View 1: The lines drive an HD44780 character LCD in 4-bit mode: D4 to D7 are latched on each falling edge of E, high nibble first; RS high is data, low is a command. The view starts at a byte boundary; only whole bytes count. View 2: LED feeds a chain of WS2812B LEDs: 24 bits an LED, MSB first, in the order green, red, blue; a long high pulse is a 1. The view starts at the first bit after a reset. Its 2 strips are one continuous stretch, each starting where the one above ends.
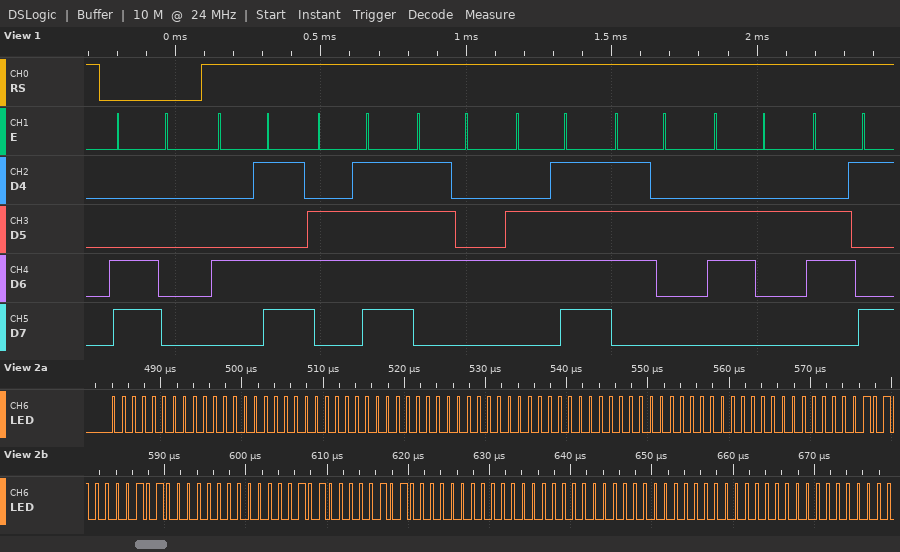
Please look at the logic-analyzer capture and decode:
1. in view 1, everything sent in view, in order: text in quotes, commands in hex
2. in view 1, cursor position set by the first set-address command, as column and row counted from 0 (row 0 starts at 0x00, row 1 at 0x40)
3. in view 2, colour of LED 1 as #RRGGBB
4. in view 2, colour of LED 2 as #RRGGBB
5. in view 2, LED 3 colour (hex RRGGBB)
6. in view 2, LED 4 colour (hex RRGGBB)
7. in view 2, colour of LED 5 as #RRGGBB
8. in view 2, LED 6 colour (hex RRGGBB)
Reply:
0xC0 "Motorbi"
column 0, row 1
#000000
#000000
#000000
#282800
#282800
#000000
